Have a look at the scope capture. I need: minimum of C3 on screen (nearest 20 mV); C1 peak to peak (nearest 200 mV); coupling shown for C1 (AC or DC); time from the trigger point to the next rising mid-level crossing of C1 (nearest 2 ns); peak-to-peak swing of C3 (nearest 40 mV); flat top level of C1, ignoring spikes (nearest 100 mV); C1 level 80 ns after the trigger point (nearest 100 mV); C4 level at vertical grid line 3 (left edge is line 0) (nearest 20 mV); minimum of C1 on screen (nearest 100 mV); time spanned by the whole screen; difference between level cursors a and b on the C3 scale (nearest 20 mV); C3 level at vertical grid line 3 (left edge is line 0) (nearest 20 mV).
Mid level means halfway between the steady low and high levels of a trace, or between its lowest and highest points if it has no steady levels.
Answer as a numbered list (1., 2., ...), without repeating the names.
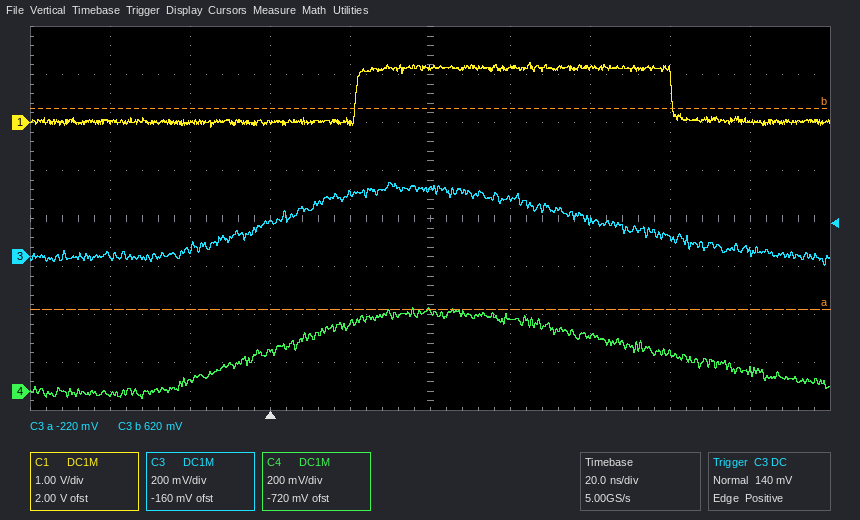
1. -40 mV
2. 1.4 V
3. DC
4. 22 ns
5. 360 mV
6. 1.1 V
7. 1.1 V
8. 160 mV
9. -100 mV
10. 200 ns
11. 840 mV
12. 140 mV
